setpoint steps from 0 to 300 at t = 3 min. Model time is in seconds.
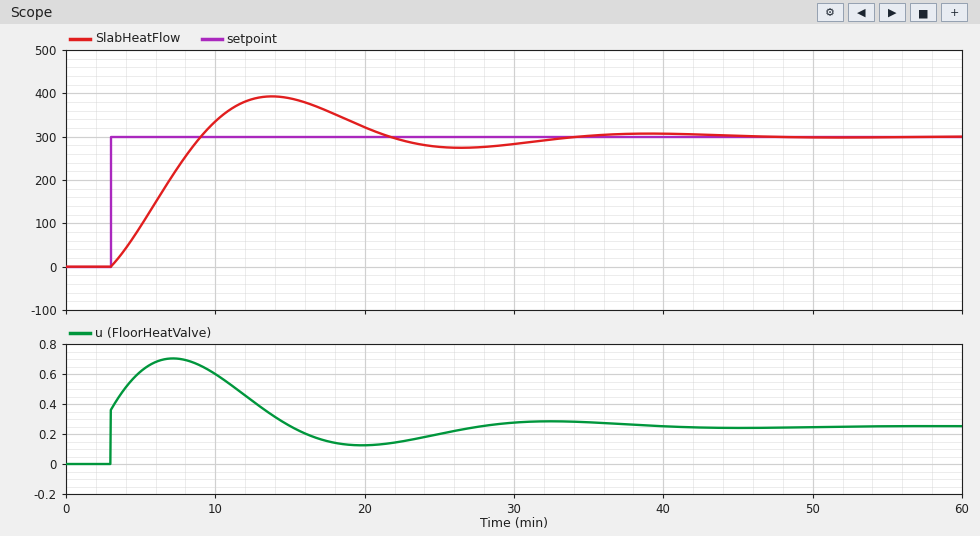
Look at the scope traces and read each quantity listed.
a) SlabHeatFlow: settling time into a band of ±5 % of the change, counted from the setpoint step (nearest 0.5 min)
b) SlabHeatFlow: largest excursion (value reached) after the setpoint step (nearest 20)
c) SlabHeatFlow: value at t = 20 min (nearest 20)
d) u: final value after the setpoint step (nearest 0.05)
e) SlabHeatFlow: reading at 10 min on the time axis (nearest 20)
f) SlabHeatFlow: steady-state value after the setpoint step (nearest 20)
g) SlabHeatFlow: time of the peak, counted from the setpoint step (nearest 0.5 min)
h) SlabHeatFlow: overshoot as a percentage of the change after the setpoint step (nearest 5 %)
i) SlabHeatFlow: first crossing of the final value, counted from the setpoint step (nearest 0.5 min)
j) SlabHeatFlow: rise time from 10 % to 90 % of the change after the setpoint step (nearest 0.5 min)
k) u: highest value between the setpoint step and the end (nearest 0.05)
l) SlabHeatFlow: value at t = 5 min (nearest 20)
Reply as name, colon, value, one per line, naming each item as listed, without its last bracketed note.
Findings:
SlabHeatFlow: settling time into a band of ±5 % of the change, counted from the setpoint step: 27.5 min
SlabHeatFlow: largest excursion (value reached) after the setpoint step: 400
SlabHeatFlow: value at t = 20 min: 320
u: final value after the setpoint step: 0.25
SlabHeatFlow: reading at 10 min on the time axis: 340
SlabHeatFlow: steady-state value after the setpoint step: 300
SlabHeatFlow: time of the peak, counted from the setpoint step: 11.0 min
SlabHeatFlow: overshoot as a percentage of the change after the setpoint step: 30 %
SlabHeatFlow: first crossing of the final value, counted from the setpoint step: 6.0 min
SlabHeatFlow: rise time from 10 % to 90 % of the change after the setpoint step: 4.5 min
u: highest value between the setpoint step and the end: 0.70
SlabHeatFlow: value at t = 5 min: 100
